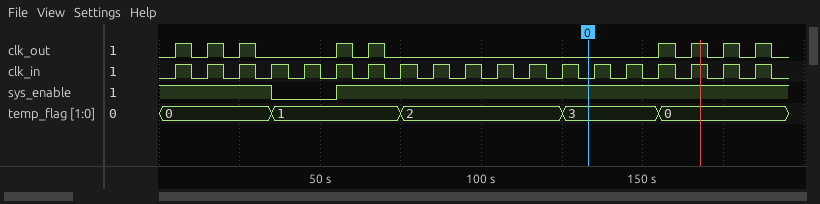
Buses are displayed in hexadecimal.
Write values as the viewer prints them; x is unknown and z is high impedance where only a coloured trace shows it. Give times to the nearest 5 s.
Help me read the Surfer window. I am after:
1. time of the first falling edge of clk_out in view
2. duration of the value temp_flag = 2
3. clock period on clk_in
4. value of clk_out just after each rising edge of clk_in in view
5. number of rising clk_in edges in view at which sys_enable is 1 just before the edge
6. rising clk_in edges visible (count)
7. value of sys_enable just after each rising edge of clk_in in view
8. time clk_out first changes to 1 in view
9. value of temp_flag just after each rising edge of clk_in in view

10 s
50 s
10 s
1 1 1 0 0 1 1 0 0 0 0 0 0 0 0 1 1 1 1
17
19
1 1 1 0 0 1 1 1 1 1 1 1 1 1 1 1 1 1 1
5 s
0, 0, 0, 1, 1, 1, 1, 2, 2, 2, 2, 2, 3, 3, 3, 0, 0, 0, 0
